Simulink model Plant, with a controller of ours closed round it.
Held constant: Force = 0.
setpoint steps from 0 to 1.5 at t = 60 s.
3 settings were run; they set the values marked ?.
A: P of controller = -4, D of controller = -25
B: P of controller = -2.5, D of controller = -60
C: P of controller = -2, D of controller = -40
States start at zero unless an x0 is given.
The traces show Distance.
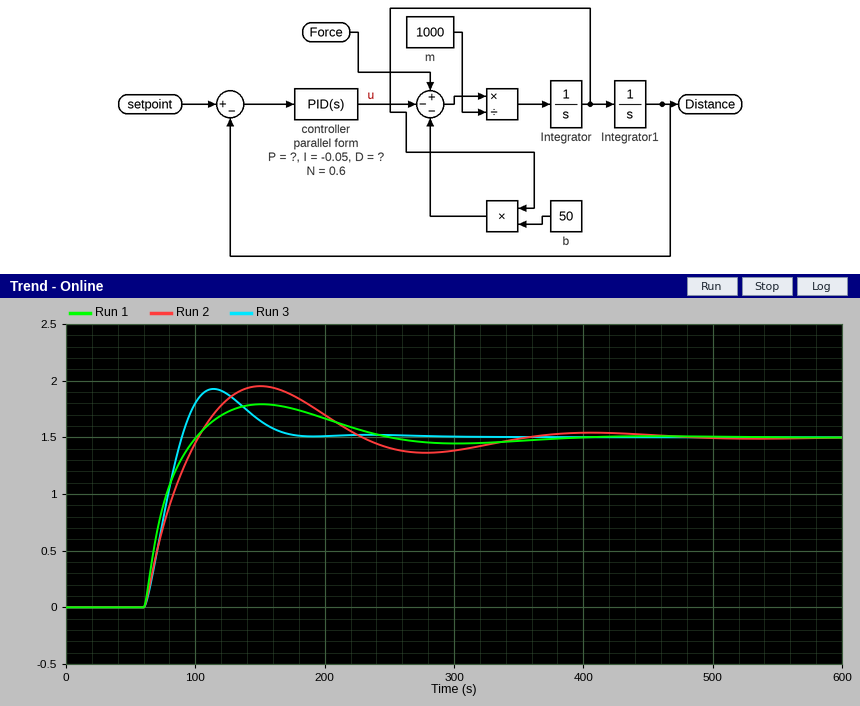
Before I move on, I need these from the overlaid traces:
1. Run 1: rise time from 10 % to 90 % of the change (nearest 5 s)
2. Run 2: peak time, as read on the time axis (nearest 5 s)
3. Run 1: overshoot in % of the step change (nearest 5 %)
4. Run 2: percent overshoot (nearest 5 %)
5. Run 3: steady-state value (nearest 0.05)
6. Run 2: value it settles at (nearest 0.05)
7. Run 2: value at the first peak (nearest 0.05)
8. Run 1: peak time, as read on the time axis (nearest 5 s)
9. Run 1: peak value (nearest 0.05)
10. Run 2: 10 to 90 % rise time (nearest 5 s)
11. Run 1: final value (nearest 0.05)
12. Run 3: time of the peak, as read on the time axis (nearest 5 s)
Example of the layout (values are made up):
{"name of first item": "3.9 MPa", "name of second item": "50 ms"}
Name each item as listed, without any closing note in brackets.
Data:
{"Run 1: rise time from 10 % to 90 % of the change": "30 s", "Run 2: peak time, as read on the time axis": "150 s", "Run 1: overshoot in % of the step change": "20 %", "Run 2: percent overshoot": "30 %", "Run 3: steady-state value": "1.50", "Run 2: value it settles at": "1.50", "Run 2: value at the first peak": "1.95", "Run 1: peak time, as read on the time axis": "150 s", "Run 1: peak value": "1.80", "Run 2: 10 to 90 % rise time": "30 s", "Run 1: final value": "1.50", "Run 3: time of the peak, as read on the time axis": "115 s"}
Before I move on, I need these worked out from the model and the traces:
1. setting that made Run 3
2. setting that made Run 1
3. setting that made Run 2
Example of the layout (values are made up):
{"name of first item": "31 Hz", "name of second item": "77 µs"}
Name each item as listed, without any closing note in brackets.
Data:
{"setting that made Run 3": "A", "setting that made Run 1": "B", "setting that made Run 2": "C"}
